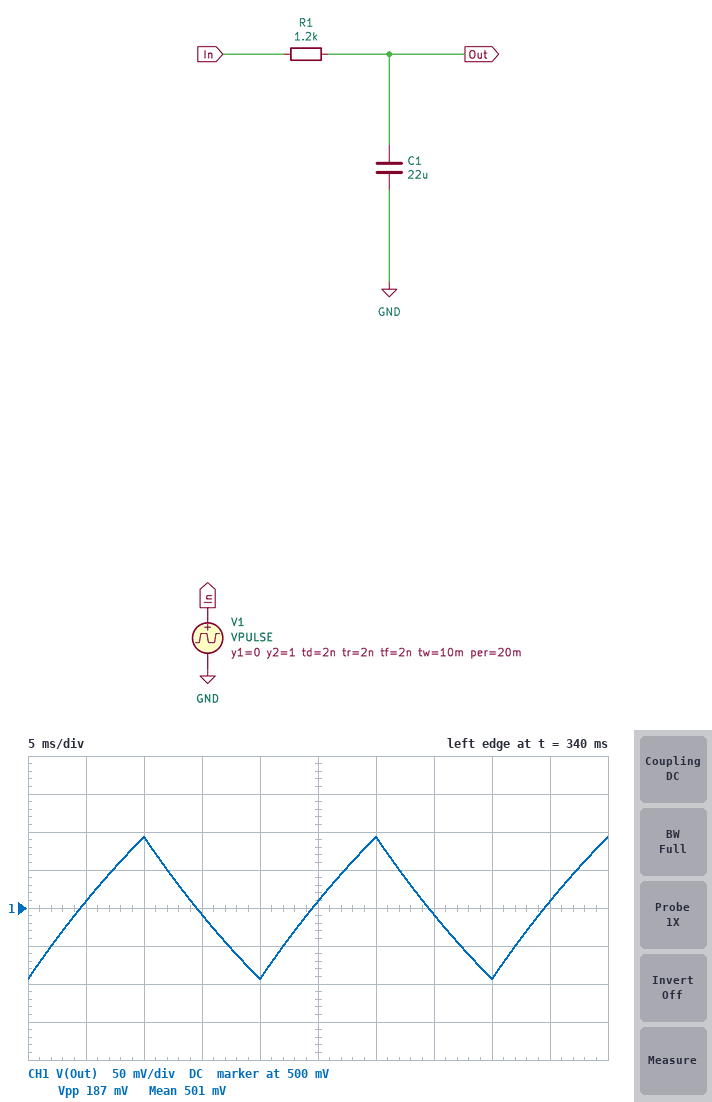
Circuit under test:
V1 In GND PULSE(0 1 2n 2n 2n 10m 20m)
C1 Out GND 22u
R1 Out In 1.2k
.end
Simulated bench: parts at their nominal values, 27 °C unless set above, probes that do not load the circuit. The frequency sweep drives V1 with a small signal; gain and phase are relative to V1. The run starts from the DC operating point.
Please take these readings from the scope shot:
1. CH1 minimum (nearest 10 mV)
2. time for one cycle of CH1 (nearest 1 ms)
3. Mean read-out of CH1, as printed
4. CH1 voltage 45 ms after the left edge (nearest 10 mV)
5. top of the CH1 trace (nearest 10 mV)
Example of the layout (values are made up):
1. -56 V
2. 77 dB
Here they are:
1. 410 mV
2. 20 ms
3. 501 mV
4. 510 mV
5. 590 mV
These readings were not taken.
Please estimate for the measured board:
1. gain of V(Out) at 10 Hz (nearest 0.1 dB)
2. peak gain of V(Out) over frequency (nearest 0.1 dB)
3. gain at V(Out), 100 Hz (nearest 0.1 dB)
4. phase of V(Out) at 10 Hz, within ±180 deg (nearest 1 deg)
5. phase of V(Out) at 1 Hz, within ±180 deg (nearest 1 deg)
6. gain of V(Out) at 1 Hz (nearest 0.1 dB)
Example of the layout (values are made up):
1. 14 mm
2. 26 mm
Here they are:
1. -5.7 dB
2. 0 dB
3. -24.4 dB
4. -59 deg
5. -9 deg
6. -0.1 dB
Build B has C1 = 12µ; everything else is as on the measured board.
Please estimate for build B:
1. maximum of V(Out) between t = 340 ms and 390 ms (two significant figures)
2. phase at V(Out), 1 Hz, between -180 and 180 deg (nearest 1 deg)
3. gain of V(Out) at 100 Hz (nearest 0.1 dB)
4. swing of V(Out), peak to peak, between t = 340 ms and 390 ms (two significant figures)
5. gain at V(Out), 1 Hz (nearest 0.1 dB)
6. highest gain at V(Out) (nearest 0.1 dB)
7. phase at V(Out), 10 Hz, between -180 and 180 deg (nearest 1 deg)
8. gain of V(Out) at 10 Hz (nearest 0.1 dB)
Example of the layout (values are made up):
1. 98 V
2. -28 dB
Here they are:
1. 670 mV
2. -5 deg
3. -19.2 dB
4. 330 mV
5. 0 dB
6. 0 dB
7. -42 deg
8. -2.6 dB
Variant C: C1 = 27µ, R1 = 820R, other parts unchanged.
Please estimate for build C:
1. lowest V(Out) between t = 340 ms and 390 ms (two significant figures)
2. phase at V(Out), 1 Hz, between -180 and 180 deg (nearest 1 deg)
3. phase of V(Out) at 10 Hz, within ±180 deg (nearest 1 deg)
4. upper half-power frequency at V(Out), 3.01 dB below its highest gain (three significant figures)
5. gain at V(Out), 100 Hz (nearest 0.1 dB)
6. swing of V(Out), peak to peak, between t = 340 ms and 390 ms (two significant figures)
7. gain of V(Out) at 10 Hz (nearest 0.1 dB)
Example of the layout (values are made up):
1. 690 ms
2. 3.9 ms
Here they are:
1. 390 mV
2. -8 deg
3. -54 deg
4. 7.19 Hz
5. -22.9 dB
6. 220 mV
7. -4.7 dB
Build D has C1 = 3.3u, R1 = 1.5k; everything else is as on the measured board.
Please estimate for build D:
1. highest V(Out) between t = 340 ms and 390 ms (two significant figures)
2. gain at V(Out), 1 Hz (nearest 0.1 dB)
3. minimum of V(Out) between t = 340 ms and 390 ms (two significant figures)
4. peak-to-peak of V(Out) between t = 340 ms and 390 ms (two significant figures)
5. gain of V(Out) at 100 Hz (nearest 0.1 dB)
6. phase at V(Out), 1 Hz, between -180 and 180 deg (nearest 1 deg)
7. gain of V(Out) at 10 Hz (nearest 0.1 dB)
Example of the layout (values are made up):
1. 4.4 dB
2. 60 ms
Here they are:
1. 880 mV
2. 0 dB
3. 120 mV
4. 770 mV
5. -10.3 dB
6. -2 deg
7. -0.4 dB
